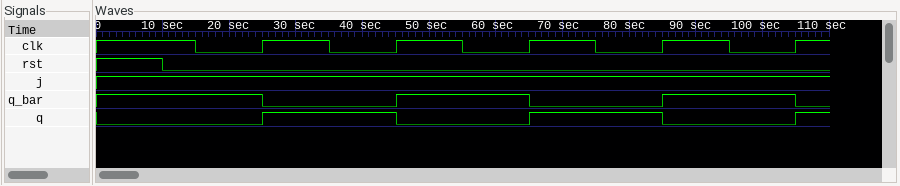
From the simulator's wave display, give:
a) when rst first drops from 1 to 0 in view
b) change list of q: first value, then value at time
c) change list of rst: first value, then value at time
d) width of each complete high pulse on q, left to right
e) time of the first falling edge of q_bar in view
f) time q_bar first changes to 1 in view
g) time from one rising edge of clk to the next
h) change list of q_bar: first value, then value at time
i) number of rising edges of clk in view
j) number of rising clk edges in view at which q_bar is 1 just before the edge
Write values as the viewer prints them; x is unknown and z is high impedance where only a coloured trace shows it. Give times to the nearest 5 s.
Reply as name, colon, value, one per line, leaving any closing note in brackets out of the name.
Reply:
when rst first drops from 1 to 0 in view: 10 s
change list of q: first value, then value at time: 0, 1 at 25 s, 0 at 45 s, 1 at 65 s, 0 at 85 s, 1 at 105 s
change list of rst: first value, then value at time: 1, 0 at 10 s
width of each complete high pulse on q, left to right: 20 s, 20 s
time of the first falling edge of q_bar in view: 25 s
time q_bar first changes to 1 in view: 45 s
time from one rising edge of clk to the next: 20 s
change list of q_bar: first value, then value at time: 1, 0 at 25 s, 1 at 45 s, 0 at 65 s, 1 at 85 s, 0 at 105 s
number of rising edges of clk in view: 5
number of rising clk edges in view at which q_bar is 1 just before the edge: 3
